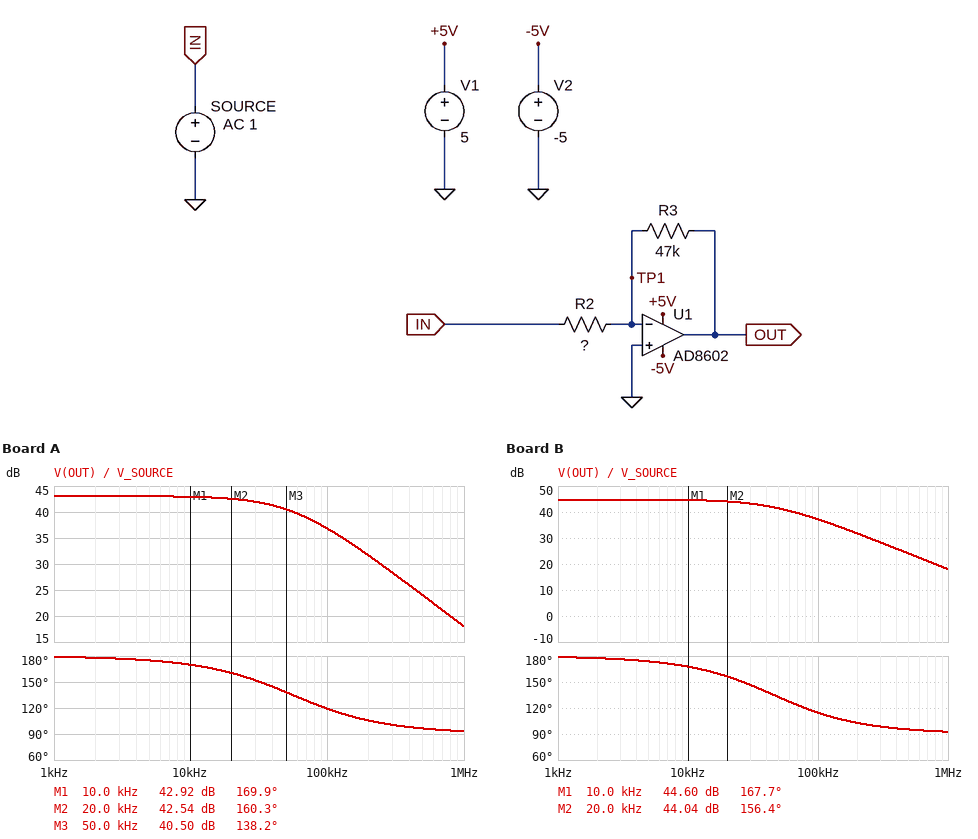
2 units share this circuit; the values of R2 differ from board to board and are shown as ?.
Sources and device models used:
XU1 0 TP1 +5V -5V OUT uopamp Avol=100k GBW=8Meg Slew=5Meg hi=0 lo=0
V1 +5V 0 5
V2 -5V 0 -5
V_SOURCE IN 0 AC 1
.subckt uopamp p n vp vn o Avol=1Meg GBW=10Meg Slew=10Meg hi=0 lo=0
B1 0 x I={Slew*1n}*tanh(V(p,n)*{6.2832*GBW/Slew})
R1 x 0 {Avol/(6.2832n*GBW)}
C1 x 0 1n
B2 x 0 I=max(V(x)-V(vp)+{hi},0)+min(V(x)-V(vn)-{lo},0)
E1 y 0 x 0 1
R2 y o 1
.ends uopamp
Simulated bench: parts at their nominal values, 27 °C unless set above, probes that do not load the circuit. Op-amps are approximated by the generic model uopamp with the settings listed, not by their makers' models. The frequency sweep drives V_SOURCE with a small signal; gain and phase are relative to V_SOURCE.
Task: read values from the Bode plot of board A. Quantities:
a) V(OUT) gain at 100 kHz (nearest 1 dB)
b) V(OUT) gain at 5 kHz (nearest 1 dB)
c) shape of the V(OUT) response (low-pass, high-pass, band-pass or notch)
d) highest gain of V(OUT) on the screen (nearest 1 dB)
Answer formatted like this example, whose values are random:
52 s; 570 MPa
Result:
37 dB; 43 dB; low-pass; 43 dB
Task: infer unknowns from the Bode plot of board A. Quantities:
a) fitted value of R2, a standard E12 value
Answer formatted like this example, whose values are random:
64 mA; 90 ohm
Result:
330 Ω
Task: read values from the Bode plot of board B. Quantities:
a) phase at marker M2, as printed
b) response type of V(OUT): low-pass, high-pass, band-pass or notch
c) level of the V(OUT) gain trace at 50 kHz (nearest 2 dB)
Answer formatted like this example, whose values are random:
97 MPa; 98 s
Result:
156.4 deg; low-pass; 42 dB
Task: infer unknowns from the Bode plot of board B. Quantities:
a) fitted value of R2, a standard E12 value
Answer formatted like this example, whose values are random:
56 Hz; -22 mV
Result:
270 Ω
